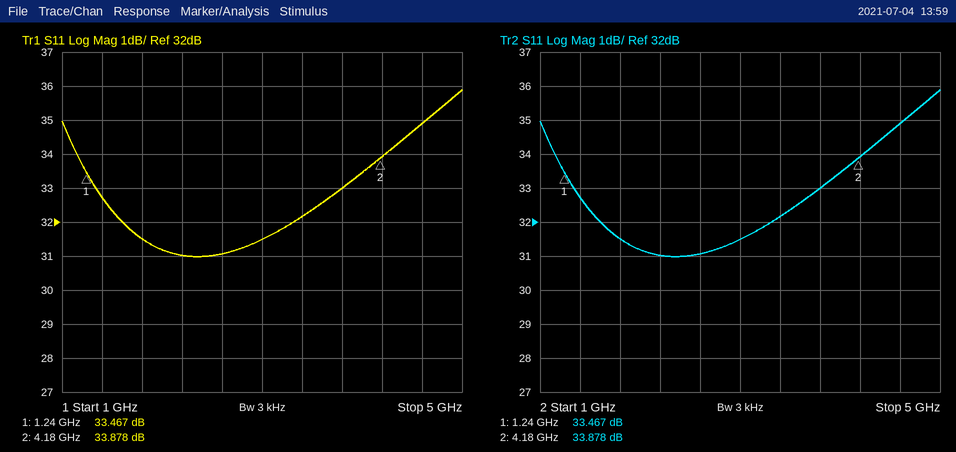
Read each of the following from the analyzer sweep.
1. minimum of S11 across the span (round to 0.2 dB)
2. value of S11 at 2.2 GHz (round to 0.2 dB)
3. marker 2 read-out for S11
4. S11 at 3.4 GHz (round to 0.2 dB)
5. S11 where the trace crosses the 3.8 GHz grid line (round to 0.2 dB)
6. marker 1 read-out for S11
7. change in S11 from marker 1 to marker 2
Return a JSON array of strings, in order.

["31.0 dB", "31.0 dB", "33.878 dB", "32.2 dB", "33.0 dB", "33.467 dB", "0.411 dB"]
